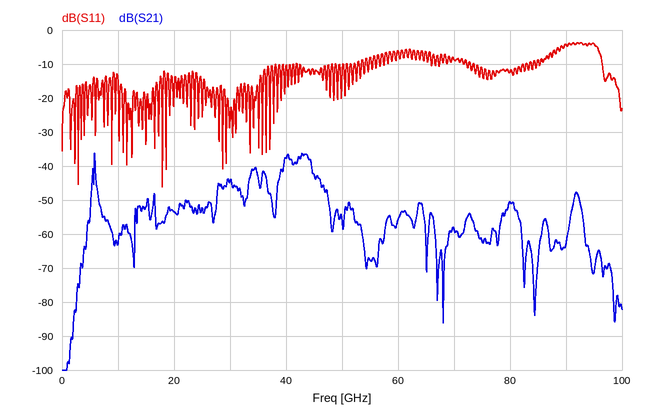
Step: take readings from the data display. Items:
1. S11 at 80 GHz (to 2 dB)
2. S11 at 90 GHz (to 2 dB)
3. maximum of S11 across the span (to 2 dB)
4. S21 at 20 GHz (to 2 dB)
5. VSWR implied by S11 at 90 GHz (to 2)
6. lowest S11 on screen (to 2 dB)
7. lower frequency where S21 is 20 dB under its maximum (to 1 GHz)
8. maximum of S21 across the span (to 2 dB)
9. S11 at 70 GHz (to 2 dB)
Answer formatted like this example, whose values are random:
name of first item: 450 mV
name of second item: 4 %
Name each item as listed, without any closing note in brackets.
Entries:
S11 at 80 GHz: -12 dB
S11 at 90 GHz: -4 dB
maximum of S11 across the span: -4 dB
S21 at 20 GHz: -54 dB
VSWR implied by S11 at 90 GHz: 4
lowest S11 on screen: -46 dB
lower frequency where S21 is 20 dB under its maximum: 5 GHz
maximum of S21 across the span: -36 dB
S11 at 70 GHz: -8 dB
